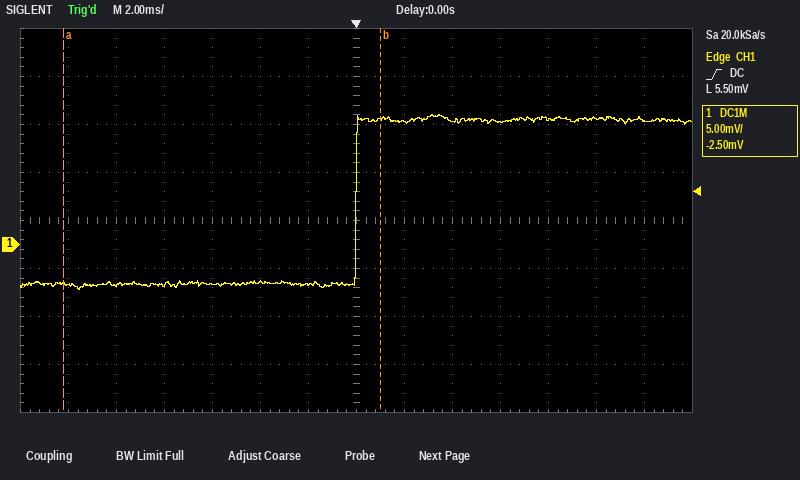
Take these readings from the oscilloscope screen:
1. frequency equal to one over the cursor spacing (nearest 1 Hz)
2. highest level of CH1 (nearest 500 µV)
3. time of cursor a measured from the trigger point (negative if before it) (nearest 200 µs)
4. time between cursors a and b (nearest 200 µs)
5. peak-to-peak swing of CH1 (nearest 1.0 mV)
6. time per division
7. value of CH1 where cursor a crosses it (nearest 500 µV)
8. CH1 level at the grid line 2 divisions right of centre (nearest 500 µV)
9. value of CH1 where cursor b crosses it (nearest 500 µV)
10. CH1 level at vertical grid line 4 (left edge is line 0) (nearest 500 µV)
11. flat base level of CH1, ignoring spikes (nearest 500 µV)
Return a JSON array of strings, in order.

["76 Hz", "13.5 mV", "-12.2 ms", "13.2 ms", "18.0 mV", "2 ms", "-4.0 mV", "13.0 mV", "13.0 mV", "-4.0 mV", "-4.0 mV"]
